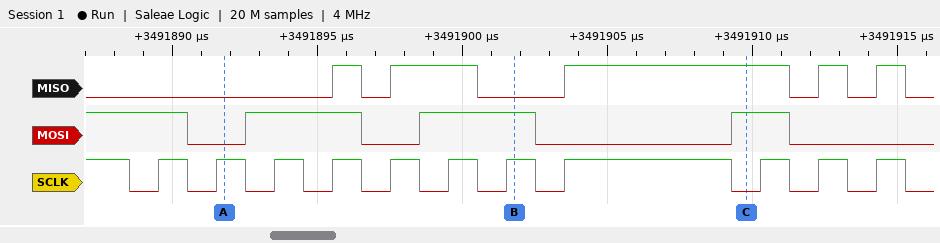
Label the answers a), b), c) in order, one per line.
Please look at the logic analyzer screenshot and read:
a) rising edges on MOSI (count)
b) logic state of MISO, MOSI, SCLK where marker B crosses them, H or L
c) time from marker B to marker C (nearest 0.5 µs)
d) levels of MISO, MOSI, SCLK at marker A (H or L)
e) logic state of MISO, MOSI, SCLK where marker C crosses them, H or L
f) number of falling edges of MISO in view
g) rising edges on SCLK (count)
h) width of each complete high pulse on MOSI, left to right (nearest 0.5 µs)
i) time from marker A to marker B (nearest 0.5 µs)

a) 3
b) MISO=L, MOSI=H, SCLK=H
c) 8 µs
d) MISO=L, MOSI=L, SCLK=H
e) MISO=H, MOSI=H, SCLK=L
f) 5
g) 11
h) 4 µs, 4 µs, 2 µs
i) 10 µs
